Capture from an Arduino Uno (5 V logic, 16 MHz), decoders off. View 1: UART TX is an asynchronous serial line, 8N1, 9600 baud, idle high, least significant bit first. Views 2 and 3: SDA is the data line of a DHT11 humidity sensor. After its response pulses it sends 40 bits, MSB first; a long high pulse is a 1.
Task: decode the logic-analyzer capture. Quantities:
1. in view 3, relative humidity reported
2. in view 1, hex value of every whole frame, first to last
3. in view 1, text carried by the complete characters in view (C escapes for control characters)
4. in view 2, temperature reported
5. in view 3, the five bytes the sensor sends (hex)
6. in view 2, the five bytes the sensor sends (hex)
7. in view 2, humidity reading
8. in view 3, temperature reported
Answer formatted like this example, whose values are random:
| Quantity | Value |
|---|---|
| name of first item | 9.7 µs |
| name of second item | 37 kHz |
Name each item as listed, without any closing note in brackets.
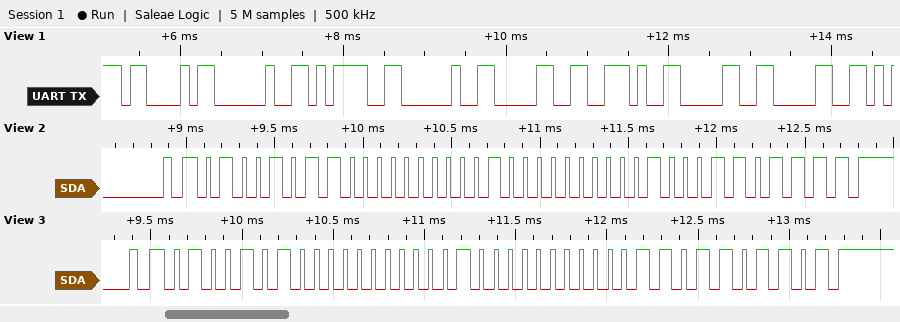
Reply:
| Quantity | Value |
|---|---|
| in view 3, relative humidity reported | 74 % |
| in view 1, hex value of every whole frame, first to last | 0x43 0x20 0x3D 0x20 0x30 0x2E 0x30 0x30 |
| in view 1, text carried by the complete characters in view | "C = 0.00" |
| in view 2, temperature reported | 32.4 °C |
| in view 3, the five bytes the sensor sends | 4A 00 20 03 6D |
| in view 2, the five bytes the sensor sends | 4B 00 20 04 6F |
| in view 2, humidity reading | 75 % |
| in view 3, temperature reported | 32.3 °C |
